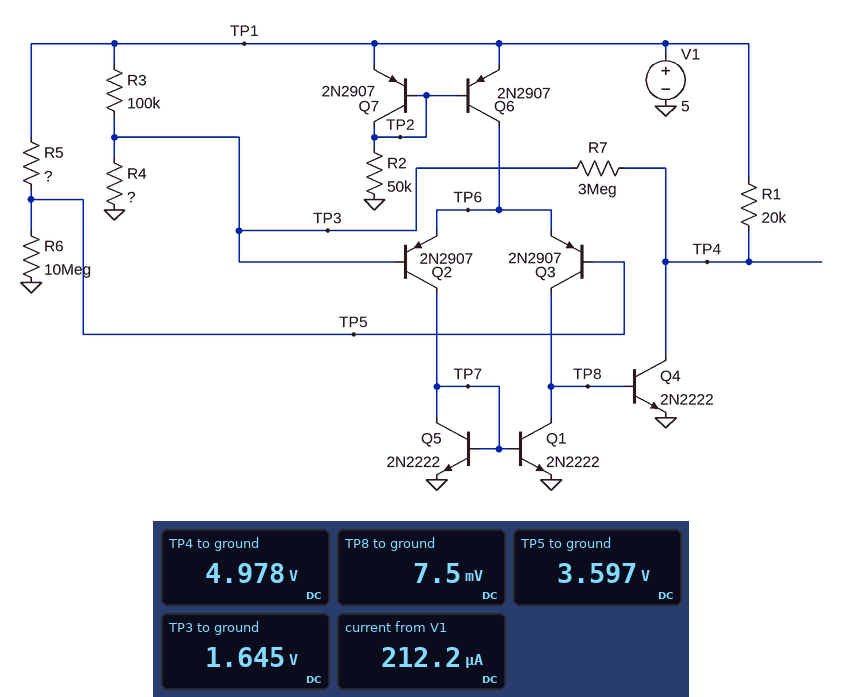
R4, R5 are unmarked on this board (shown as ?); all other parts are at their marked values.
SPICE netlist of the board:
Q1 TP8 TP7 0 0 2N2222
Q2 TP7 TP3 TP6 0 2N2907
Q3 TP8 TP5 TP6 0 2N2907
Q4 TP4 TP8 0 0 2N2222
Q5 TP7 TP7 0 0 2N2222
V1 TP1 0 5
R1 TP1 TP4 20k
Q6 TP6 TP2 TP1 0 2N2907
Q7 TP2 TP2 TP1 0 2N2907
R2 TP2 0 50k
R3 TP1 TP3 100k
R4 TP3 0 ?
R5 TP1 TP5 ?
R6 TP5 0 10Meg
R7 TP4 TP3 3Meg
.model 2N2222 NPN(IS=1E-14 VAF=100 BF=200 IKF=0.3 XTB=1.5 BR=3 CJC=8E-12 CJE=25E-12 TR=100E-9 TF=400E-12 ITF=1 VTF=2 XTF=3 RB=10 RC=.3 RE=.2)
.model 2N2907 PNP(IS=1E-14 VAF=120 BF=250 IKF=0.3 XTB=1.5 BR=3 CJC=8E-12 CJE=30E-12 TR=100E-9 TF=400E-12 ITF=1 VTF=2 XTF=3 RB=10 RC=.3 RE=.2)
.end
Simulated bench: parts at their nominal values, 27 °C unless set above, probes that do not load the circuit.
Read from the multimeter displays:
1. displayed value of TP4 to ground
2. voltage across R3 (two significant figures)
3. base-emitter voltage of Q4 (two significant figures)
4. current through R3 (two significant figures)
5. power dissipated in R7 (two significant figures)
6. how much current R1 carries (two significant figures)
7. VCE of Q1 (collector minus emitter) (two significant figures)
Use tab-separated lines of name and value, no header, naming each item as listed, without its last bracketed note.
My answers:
displayed value of TP4 to ground	4.978 V
voltage across R3	3.4 V
base-emitter voltage of Q4	7.5 mV
current through R3	34 µA
power dissipated in R7	3.7 µW
how much current R1 carries	1.1 µA
VCE of Q1 (collector minus emitter)	7.5 mV
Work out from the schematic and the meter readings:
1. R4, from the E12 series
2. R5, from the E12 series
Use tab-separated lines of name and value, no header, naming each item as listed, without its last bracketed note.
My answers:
R4, from the E12 series	47 kΩ
R5, from the E12 series	3.9 MΩ
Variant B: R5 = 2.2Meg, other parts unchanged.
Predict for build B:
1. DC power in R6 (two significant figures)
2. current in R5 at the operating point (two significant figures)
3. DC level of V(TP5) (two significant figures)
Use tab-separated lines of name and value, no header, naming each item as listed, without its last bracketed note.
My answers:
DC power in R6	1.7 µW
current in R5 at the operating point	410 nA
DC level of V(TP5)	4.1 V
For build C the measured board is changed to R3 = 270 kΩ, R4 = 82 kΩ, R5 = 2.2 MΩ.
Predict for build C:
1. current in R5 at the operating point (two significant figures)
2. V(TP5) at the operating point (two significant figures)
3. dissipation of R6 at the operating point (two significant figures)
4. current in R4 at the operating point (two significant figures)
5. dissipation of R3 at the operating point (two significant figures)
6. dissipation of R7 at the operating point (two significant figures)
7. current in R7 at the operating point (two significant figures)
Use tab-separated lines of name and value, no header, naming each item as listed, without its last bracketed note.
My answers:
current in R5 at the operating point	410 nA
V(TP5) at the operating point	4.1 V
dissipation of R6 at the operating point	1.7 µW
current in R4 at the operating point	15 µA
dissipation of R3 at the operating point	52 µW
dissipation of R7 at the operating point	4.6 µW
current in R7 at the operating point	1.2 µA
